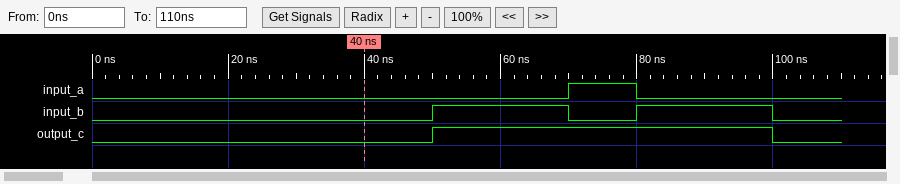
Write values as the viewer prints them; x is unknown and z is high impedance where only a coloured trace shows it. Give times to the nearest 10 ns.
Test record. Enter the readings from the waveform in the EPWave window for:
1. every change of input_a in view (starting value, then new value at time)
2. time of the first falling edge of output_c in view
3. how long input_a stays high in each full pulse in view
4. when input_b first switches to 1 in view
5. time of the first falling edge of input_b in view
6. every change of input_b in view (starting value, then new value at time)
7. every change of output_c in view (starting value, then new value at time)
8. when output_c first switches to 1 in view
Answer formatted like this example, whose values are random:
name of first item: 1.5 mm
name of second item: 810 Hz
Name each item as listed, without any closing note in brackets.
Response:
every change of input_a in view: 0, 1 at 70 ns, 0 at 80 ns
time of the first falling edge of output_c in view: 100 ns
how long input_a stays high in each full pulse in view: 10 ns
when input_b first switches to 1 in view: 50 ns
time of the first falling edge of input_b in view: 70 ns
every change of input_b in view: 0, 1 at 50 ns, 0 at 70 ns, 1 at 80 ns, 0 at 100 ns
every change of output_c in view: 0, 1 at 50 ns, 0 at 100 ns
when output_c first switches to 1 in view: 50 ns
